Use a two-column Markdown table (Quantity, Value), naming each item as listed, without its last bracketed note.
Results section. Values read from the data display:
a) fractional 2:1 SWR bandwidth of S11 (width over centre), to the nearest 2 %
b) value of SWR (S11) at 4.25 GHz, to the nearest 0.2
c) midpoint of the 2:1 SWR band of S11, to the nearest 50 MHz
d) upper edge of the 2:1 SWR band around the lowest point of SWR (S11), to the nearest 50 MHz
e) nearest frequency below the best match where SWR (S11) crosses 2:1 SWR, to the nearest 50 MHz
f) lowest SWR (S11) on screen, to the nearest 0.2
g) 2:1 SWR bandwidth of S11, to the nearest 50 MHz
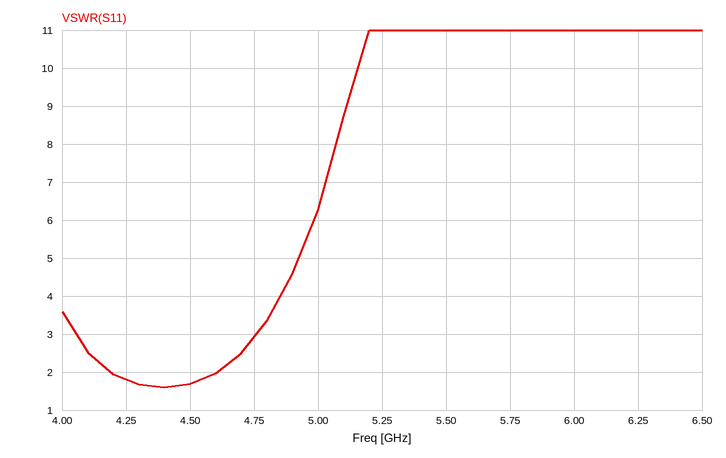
| Quantity | Value |
|---|---|
| fractional 2:1 SWR bandwidth of S11 (width over centre), to the nearest 2 % | 10 % |
| value of SWR (S11) at 4.25 GHz, to the nearest 0.2 | 1.8 |
| midpoint of the 2:1 SWR band of S11, to the nearest 50 MHz | 4.40 GHz |
| upper edge of the 2:1 SWR band around the lowest point of SWR (S11), to the nearest 50 MHz | 4.60 GHz |
| nearest frequency below the best match where SWR (S11) crosses 2:1 SWR, to the nearest 50 MHz | 4.20 GHz |
| lowest SWR (S11) on screen, to the nearest 0.2 | 1.6 |
| 2:1 SWR bandwidth of S11, to the nearest 50 MHz | 400 MHz |
